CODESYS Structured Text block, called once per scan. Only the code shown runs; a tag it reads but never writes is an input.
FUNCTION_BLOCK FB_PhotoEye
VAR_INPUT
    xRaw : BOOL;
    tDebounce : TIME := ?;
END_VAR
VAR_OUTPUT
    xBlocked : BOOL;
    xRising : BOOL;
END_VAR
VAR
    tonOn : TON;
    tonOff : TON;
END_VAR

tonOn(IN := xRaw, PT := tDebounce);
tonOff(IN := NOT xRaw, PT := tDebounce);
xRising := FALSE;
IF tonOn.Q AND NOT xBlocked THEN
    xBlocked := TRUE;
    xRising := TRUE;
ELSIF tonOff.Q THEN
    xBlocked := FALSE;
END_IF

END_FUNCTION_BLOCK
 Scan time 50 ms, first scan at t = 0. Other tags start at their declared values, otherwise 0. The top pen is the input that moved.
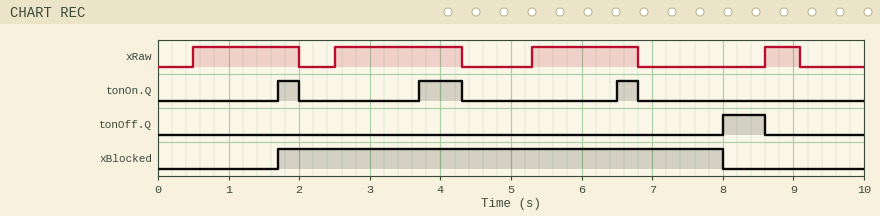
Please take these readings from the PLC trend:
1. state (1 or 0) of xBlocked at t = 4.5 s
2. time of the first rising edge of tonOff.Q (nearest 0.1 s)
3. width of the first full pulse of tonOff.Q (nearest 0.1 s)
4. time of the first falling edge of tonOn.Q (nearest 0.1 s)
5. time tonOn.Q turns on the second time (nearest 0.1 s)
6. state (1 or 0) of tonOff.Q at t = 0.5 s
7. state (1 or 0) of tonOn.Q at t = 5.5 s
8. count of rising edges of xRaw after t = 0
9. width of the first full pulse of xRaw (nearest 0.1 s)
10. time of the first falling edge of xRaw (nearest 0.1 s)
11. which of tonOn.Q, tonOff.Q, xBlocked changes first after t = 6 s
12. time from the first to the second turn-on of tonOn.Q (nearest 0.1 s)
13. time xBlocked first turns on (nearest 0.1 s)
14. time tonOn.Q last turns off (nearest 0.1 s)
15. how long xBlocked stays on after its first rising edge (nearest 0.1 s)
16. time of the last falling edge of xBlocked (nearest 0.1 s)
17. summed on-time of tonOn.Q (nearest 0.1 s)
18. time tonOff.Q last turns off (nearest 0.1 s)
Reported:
1
8.0 s
0.6 s
2.0 s
3.7 s
0
0
4
1.5 s
2.0 s
tonOn.Q
2.0 s
1.7 s
6.8 s
6.3 s
8.0 s
1.2 s
8.6 s
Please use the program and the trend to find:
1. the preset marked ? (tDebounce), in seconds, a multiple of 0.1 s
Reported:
1.2 s
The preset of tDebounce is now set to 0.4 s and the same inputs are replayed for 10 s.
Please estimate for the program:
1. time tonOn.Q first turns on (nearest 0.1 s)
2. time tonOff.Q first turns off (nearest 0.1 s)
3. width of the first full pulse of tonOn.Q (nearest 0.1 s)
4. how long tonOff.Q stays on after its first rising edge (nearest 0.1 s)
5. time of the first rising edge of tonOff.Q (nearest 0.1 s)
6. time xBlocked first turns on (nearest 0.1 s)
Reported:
0.9 s
0.5 s
1.1 s
0.1 s
0.4 s
0.9 s
